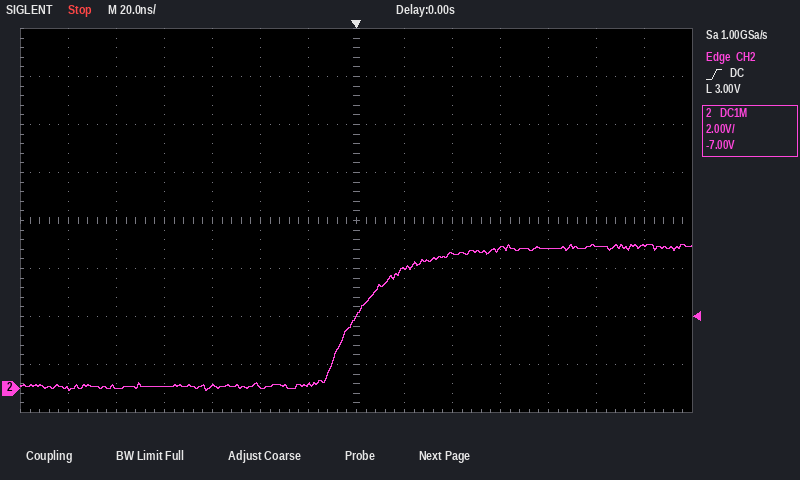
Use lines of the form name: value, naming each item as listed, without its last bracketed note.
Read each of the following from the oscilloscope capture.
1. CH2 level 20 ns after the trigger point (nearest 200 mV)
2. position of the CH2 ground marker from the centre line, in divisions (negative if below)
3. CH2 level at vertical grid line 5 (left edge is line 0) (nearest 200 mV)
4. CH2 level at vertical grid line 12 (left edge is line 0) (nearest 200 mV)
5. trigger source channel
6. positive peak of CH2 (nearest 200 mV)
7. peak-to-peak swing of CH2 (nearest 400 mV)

CH2 level 20 ns after the trigger point: 5.0 V
position of the CH2 ground marker from the centre line, in divisions: -3.5 div
CH2 level at vertical grid line 5 (left edge is line 0): 0.0 V
CH2 level at vertical grid line 12 (left edge is line 0): 6.0 V
trigger source channel: CH2
positive peak of CH2: 6.0 V
peak-to-peak swing of CH2: 6.0 V
